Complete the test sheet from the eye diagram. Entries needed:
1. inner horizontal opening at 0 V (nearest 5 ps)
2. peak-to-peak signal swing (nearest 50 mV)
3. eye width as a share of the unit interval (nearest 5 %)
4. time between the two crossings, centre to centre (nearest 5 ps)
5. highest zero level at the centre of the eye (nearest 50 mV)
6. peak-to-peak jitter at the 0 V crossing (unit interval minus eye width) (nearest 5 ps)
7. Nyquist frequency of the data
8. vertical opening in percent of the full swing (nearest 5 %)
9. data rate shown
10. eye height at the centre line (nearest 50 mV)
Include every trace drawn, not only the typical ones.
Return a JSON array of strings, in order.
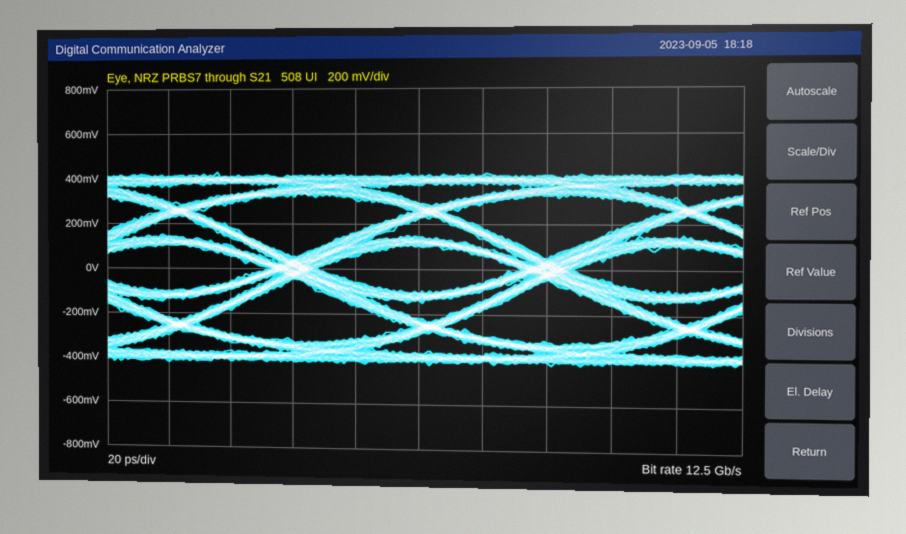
["65 ps", "850 mV", "80 %", "80 ps", "-100 mV", "15 ps", "6.25 GHz", "25 %", "12.5 Gb/s", "200 mV"]
